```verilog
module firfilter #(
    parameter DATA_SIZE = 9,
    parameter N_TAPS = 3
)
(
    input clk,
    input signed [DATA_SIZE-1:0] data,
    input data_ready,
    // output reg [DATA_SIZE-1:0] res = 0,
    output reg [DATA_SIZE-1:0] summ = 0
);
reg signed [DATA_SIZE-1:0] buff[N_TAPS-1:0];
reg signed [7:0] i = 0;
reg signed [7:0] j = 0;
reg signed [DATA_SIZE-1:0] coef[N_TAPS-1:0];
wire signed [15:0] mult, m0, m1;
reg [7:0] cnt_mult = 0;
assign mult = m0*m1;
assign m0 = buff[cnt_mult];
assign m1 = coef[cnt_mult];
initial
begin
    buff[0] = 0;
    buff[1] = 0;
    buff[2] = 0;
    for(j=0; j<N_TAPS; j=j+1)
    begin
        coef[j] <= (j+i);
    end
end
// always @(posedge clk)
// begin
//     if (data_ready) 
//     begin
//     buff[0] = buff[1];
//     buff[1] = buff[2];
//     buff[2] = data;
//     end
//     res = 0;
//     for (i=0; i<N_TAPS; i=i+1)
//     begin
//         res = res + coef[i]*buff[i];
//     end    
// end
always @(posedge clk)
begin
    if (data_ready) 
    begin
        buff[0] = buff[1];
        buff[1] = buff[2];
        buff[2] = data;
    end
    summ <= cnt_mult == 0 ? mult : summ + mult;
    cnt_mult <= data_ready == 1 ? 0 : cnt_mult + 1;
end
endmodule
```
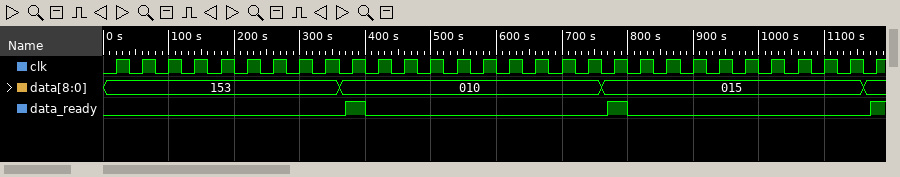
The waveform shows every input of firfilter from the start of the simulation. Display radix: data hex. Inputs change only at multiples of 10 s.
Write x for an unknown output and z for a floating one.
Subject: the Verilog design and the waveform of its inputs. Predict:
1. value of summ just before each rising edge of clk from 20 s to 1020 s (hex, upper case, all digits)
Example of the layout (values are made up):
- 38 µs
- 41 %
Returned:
- 000, 000, 000, 000, x, x, x, x, x, x, x, 000, 000, 020, x, x, x, x, x, x, x, 000, 010, 03A, x, x
